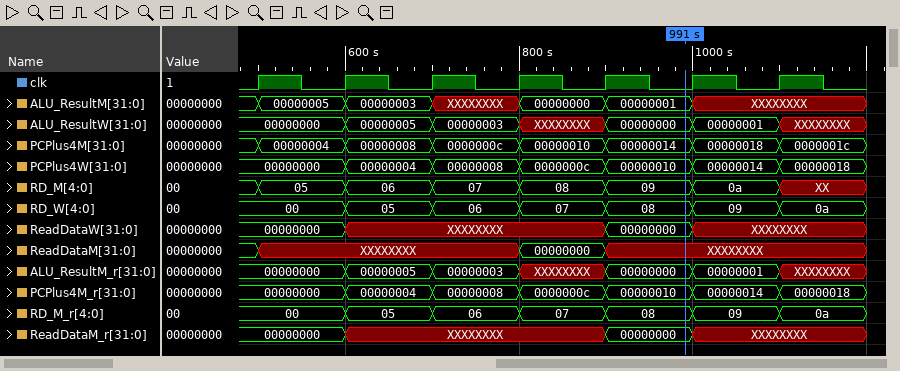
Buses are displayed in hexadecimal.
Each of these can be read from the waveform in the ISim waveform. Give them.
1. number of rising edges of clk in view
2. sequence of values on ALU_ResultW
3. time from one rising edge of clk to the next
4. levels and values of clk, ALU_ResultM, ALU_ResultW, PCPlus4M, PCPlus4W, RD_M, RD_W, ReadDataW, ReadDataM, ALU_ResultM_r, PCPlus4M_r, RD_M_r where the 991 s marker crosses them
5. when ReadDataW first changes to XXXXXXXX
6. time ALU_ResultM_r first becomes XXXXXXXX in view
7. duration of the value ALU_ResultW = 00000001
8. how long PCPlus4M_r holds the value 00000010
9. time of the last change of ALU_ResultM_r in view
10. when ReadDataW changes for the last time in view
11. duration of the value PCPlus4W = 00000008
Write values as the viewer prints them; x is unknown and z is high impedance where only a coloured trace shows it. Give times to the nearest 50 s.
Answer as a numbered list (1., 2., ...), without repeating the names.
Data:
1. 7
2. 00000000, 00000005, 00000003, XXXXXXXX, 00000000, 00000001, XXXXXXXX
3. 100 s
4. clk=0, ALU_ResultM=00000001, ALU_ResultW=00000000, PCPlus4M=00000014, PCPlus4W=00000010, RD_M=09, RD_W=08, ReadDataW=00000000, ReadDataM=XXXXXXXX, ALU_ResultM_r=00000000, PCPlus4M_r=00000010, RD_M_r=08
5. 600 s
6. 800 s
7. 100 s
8. 100 s
9. 1100 s
10. 1000 s
11. 100 s
